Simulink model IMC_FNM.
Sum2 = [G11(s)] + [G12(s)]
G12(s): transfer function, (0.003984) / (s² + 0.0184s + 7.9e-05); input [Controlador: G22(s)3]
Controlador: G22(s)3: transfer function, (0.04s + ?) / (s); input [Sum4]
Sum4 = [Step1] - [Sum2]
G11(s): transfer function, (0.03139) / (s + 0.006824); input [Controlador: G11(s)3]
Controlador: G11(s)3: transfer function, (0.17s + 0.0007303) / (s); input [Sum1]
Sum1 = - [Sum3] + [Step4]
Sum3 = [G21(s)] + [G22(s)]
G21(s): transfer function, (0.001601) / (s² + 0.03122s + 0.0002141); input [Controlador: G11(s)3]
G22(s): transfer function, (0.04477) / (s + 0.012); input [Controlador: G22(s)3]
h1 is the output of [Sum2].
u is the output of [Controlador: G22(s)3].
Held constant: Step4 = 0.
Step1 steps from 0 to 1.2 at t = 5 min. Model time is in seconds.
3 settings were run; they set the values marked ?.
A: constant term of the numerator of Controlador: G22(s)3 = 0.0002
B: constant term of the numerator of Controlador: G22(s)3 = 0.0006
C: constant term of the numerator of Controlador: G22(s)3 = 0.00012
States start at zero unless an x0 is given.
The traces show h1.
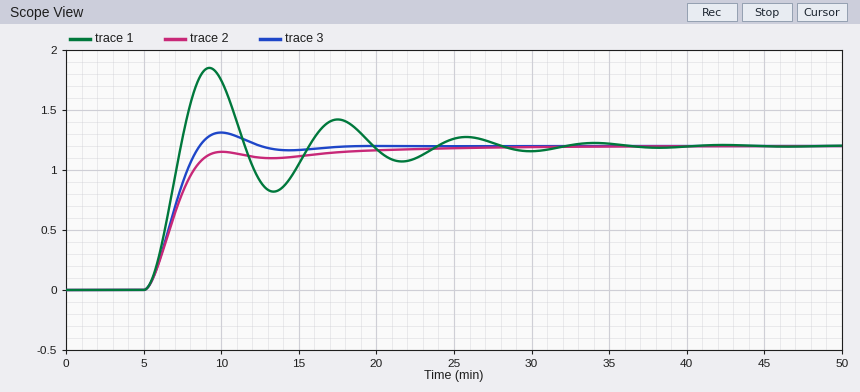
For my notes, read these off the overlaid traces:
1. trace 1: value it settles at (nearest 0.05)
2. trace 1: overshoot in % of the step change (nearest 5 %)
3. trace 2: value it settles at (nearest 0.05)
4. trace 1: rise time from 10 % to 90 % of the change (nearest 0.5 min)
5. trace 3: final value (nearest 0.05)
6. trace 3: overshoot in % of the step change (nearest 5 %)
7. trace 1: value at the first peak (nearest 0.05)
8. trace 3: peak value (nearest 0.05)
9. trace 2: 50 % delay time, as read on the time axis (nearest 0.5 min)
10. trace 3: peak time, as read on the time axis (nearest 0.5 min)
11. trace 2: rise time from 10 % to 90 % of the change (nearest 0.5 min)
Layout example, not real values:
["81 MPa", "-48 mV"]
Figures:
["1.20", "55 %", "1.20", "1.5 min", "1.20", "10 %", "1.85", "1.30", "7.0 min", "10.0 min", "3.0 min"]
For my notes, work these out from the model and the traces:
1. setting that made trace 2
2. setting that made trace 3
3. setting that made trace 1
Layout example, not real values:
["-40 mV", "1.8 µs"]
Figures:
["C", "A", "B"]
